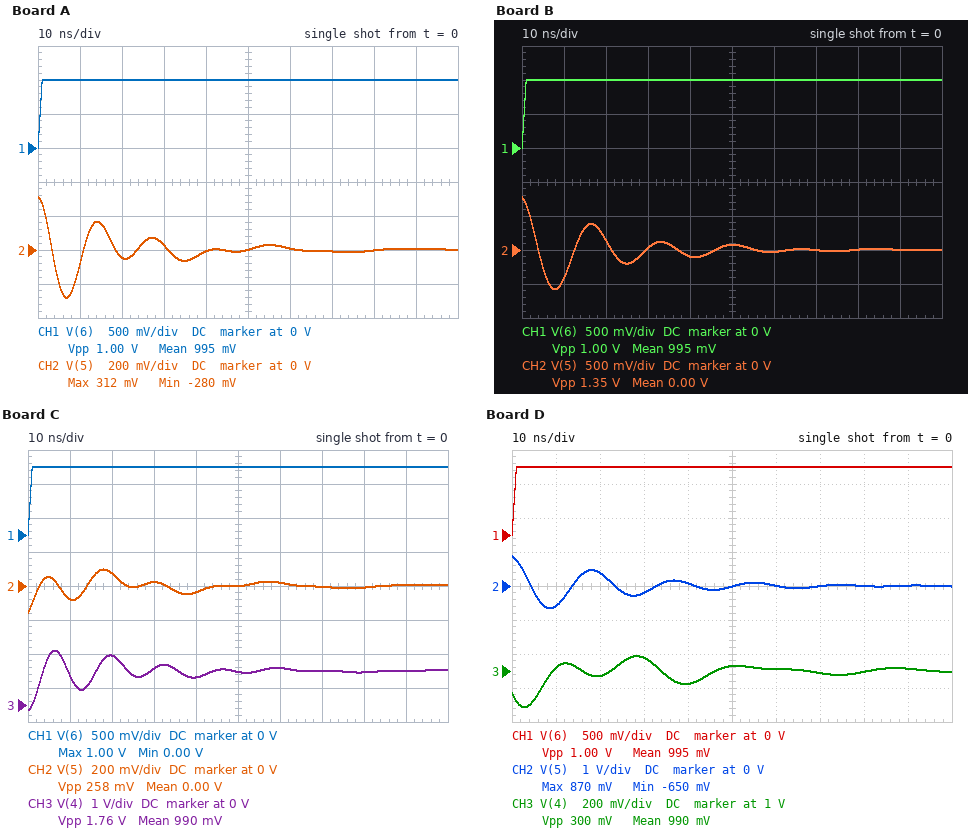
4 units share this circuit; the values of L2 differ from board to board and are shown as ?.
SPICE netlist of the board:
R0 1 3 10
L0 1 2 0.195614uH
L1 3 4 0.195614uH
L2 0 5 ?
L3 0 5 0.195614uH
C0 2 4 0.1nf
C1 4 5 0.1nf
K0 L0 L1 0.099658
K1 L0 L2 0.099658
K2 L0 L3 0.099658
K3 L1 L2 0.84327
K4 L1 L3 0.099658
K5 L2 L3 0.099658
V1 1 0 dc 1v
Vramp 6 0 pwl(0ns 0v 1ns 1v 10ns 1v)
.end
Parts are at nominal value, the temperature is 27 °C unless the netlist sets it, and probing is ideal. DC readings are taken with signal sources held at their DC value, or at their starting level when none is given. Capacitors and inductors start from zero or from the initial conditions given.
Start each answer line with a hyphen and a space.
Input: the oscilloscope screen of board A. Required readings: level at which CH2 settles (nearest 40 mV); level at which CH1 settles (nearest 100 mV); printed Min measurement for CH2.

- 0 V
- 1.0 V
- -280 mV
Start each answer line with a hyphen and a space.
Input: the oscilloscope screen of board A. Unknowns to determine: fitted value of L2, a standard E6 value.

- 150 nH
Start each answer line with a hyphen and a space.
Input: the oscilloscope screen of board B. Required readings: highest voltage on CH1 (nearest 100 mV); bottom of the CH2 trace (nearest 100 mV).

- 1.0 V
- -600 mV
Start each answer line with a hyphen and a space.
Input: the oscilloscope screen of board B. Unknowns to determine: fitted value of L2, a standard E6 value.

- 330 nH
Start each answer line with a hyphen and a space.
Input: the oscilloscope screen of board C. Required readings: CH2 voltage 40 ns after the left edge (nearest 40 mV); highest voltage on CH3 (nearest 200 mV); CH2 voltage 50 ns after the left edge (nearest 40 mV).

- -40 mV
- 1.6 V
- 0 V
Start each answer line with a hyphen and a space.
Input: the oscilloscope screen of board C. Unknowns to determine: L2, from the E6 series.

- 68 nH
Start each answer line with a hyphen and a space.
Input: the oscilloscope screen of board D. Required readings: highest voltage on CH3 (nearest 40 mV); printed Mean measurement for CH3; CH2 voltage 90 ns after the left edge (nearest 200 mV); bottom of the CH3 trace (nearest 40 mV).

- 1.08 V
- 990 mV
- 0 V
- 800 mV
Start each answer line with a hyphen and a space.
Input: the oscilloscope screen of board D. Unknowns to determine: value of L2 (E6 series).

- 470 nH
